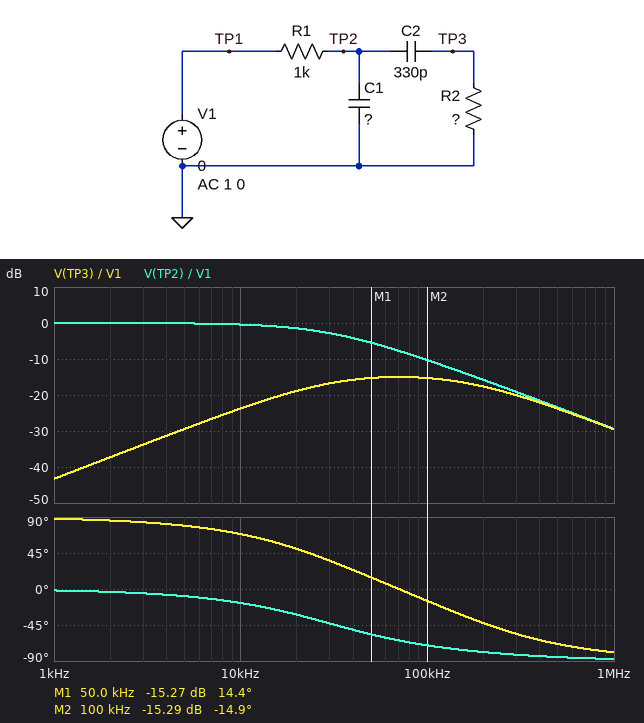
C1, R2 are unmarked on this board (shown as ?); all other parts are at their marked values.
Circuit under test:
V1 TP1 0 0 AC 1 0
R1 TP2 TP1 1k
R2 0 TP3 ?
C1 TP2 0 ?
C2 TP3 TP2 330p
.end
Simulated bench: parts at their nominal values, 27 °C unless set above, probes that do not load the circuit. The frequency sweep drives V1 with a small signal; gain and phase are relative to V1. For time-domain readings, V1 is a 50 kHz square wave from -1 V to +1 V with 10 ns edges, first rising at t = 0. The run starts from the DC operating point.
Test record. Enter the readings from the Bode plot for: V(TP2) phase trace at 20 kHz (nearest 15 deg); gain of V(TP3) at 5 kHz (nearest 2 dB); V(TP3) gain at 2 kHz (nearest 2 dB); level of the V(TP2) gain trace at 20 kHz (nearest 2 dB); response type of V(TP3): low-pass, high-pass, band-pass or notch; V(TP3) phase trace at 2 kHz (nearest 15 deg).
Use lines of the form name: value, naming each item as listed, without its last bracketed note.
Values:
V(TP2) phase trace at 20 kHz: -30 deg
gain of V(TP3) at 5 kHz: -30 dB
V(TP3) gain at 2 kHz: -38 dB
level of the V(TP2) gain trace at 20 kHz: -2 dB
response type of V(TP3): low-pass, high-pass, band-pass or notch: band-pass
V(TP3) phase trace at 2 kHz: 90 deg
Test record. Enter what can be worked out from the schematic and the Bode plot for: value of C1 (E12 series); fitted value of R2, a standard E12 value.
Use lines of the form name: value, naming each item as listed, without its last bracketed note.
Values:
value of C1: 4.7 nF
fitted value of R2, a standard E12 value: 3.3 kΩ
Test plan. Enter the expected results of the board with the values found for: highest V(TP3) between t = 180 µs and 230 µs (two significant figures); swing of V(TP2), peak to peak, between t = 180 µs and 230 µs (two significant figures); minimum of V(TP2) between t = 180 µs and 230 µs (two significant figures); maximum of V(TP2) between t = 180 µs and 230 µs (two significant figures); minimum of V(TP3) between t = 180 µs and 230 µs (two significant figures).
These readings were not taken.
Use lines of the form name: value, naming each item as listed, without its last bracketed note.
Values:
highest V(TP3) between t = 180 µs and 230 µs: 240 mV
swing of V(TP2), peak to peak, between t = 180 µs and 230 µs: 1.5 V
minimum of V(TP2) between t = 180 µs and 230 µs: -760 mV
maximum of V(TP2) between t = 180 µs and 230 µs: 760 mV
minimum of V(TP3) between t = 180 µs and 230 µs: -240 mV
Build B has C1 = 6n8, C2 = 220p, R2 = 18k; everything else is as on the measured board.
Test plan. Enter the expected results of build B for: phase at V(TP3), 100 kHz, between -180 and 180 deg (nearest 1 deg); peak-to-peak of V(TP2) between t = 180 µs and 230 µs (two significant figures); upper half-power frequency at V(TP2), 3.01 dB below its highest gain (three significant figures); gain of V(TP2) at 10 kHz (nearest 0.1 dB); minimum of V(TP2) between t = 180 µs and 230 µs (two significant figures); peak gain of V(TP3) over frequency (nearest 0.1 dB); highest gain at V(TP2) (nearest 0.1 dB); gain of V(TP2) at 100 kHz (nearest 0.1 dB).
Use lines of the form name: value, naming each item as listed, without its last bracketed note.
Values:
phase at V(TP3), 100 kHz, between -180 and 180 deg: -54 deg
peak-to-peak of V(TP2) between t = 180 µs and 230 µs: 1.2 V
upper half-power frequency at V(TP2), 3.01 dB below its highest gain: 22.5 kHz
gain of V(TP2) at 10 kHz: -0.8 dB
minimum of V(TP2) between t = 180 µs and 230 µs: -620 mV
peak gain of V(TP3) over frequency: -8.9 dB
highest gain at V(TP2): 0 dB
gain of V(TP2) at 100 kHz: -12.9 dB
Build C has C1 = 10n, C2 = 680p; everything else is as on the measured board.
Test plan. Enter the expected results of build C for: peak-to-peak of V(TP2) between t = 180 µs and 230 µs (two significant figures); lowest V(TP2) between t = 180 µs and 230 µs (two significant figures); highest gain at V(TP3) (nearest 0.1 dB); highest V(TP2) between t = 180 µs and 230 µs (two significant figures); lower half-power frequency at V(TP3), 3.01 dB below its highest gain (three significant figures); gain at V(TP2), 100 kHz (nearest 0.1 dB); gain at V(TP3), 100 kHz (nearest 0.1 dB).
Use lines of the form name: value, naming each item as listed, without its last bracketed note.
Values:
peak-to-peak of V(TP2) between t = 180 µs and 230 µs: 880 mV
lowest V(TP2) between t = 180 µs and 230 µs: -440 mV
highest gain at V(TP3): -15.2 dB
highest V(TP2) between t = 180 µs and 230 µs: 440 mV
lower half-power frequency at V(TP3), 3.01 dB below its highest gain: 11.0 kHz
gain at V(TP2), 100 kHz: -16.3 dB
gain at V(TP3), 100 kHz: -18.1 dB
